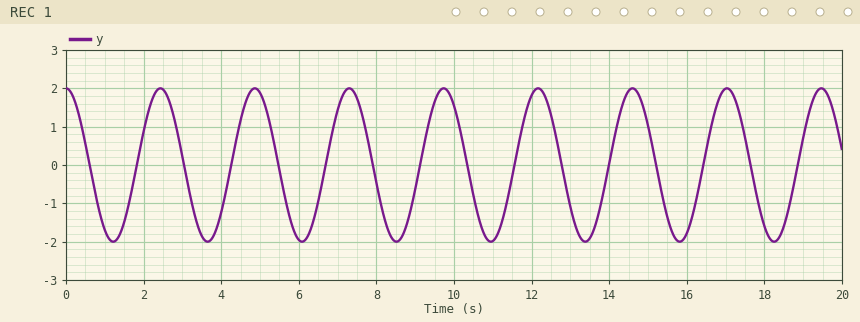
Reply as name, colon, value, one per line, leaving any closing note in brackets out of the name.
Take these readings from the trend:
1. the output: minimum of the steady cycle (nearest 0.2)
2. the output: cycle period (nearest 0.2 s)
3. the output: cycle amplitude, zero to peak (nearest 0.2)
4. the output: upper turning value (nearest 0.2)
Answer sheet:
the output: minimum of the steady cycle: -2.0
the output: cycle period: 2.4 s
the output: cycle amplitude, zero to peak: 2.0
the output: upper turning value: 2.0
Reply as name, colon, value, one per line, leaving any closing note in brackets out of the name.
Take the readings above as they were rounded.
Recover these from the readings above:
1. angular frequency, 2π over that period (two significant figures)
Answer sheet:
angular frequency, 2π over that period: 2.6 rad/s
